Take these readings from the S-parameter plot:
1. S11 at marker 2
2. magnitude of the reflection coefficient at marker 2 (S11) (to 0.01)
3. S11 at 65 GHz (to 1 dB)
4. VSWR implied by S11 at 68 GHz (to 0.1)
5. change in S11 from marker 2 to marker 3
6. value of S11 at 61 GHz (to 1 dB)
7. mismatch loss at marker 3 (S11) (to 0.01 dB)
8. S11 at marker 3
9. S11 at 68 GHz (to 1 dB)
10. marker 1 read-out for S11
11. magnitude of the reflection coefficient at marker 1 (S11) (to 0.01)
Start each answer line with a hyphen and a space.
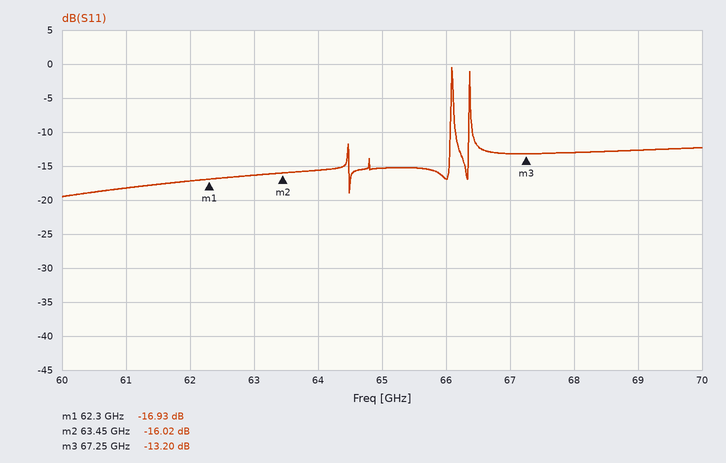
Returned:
- -16.02 dB
- 0.16
- -15 dB
- 1.6
- 2.82 dB
- -18 dB
- 0.21 dB
- -13.20 dB
- -13 dB
- -16.93 dB
- 0.14
